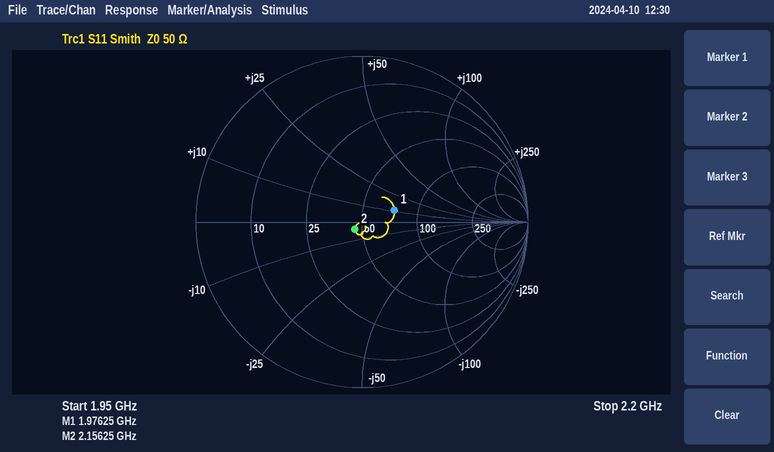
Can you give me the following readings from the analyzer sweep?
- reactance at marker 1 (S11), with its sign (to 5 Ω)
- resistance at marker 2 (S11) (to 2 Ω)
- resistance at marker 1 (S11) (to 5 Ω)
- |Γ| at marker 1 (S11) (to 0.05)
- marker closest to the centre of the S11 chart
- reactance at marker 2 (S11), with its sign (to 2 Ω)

+10 Ω
46 Ω
75 Ω
0.20
marker 2
-4 Ω
